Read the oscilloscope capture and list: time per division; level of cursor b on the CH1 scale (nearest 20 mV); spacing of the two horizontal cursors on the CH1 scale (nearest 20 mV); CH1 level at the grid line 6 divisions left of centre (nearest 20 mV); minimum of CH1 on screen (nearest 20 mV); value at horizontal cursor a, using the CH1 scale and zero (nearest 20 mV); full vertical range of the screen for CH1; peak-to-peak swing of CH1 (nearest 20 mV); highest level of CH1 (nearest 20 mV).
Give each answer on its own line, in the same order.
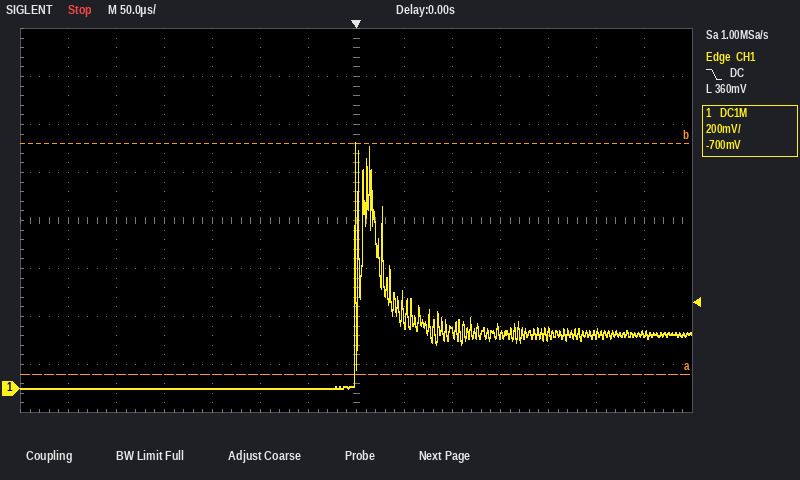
50 µs
1.02 V
960 mV
0 mV
0 mV
60 mV
1.6 V
1.02 V
1.02 V
